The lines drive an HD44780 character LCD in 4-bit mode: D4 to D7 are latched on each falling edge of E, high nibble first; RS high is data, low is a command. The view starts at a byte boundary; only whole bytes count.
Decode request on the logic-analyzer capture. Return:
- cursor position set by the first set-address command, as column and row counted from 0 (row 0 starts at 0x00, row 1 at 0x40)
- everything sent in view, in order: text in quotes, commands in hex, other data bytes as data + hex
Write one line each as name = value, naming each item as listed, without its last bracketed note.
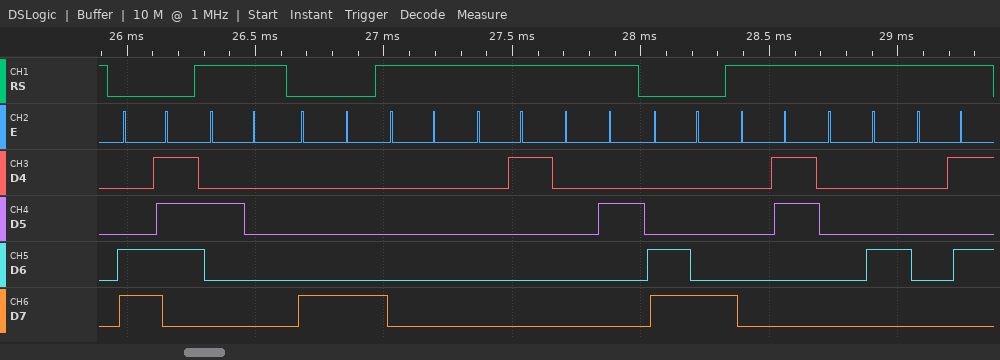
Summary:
cursor position set by the first set-address command, as column and row counted from 0 = column 7, row 1
everything sent in view, in order: text in quotes, commands in hex, other data bytes as data + hex = 0xC7 " " 0x88 data 00 01 02 0xC8 data 03 04 05
